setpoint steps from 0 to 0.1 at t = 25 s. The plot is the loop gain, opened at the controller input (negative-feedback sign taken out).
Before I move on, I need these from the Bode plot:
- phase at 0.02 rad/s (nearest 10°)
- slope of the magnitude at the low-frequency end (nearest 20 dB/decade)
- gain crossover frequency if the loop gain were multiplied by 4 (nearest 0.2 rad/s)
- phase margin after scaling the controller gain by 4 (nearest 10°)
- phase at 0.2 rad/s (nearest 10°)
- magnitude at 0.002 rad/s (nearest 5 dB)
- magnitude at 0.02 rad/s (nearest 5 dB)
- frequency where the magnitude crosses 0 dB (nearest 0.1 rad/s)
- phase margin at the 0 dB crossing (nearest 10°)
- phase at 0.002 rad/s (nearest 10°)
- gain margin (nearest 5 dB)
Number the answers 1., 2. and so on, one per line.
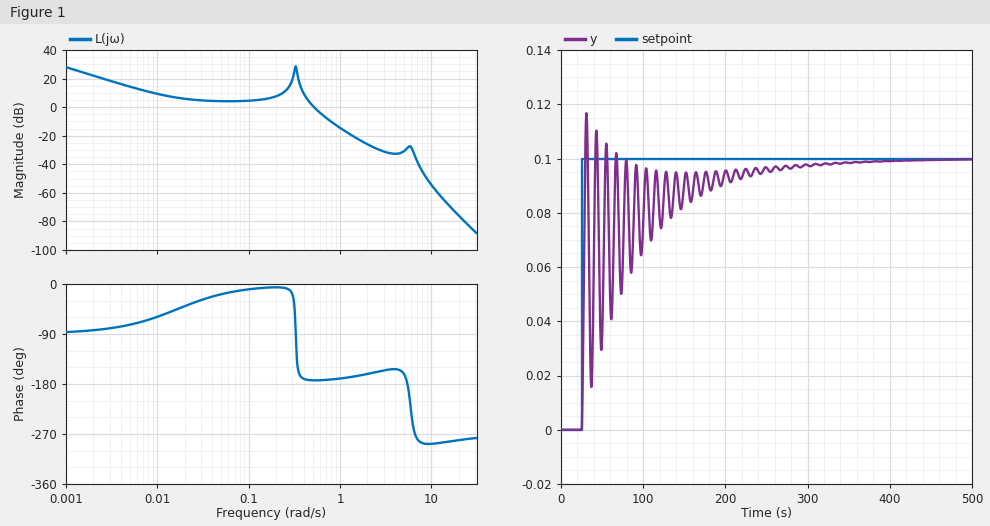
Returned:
1. -40°
2. -20 dB/decade
3. 0.8 rad/s
4. 10°
5. -10°
6. 20 dB
7. 5 dB
8. 0.5 rad/s
9. 10°
10. -80°
11. 30 dB
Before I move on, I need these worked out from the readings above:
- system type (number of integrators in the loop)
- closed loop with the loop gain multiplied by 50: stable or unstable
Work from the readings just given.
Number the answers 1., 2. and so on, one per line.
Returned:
1. 1
2. unstable
